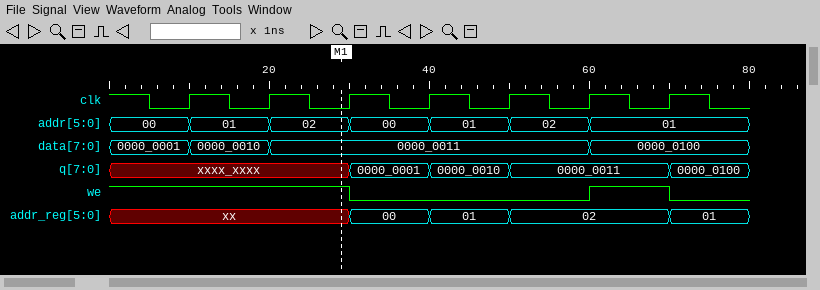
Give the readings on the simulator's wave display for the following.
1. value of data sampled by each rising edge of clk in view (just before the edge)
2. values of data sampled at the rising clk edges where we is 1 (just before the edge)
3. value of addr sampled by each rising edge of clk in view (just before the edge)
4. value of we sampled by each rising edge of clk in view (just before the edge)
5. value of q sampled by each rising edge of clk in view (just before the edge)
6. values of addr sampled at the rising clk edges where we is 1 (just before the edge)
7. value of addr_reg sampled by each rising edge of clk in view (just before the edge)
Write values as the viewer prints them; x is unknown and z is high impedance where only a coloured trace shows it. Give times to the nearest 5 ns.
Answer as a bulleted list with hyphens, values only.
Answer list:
- 0000_0001, 0000_0010, 0000_0011, 0000_0011, 0000_0011, 0000_0011, 0000_0100
- 0000_0001, 0000_0010, 0000_0011, 0000_0100
- 00, 01, 02, 00, 01, 02, 01
- 1 1 1 0 0 0 1
- xxxx_xxxx, xxxx_xxxx, xxxx_xxxx, 0000_0001, 0000_0010, 0000_0011, 0000_0011
- 00, 01, 02, 01
- xx, xx, xx, 00, 01, 02, 02
